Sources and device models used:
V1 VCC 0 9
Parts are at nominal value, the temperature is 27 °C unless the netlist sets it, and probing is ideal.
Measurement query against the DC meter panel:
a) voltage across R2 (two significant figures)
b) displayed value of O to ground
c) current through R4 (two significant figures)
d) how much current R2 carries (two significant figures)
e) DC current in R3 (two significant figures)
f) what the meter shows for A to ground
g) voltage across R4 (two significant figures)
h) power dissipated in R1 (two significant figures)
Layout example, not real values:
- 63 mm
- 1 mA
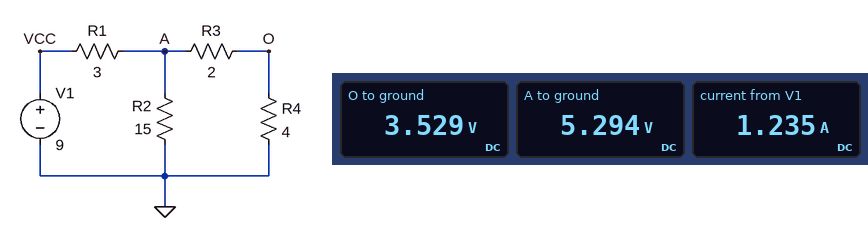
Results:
- 5.3 V
- 3.529 V
- 880 mA
- 350 mA
- 880 mA
- 5.294 V
- 3.5 V
- 4.6 W
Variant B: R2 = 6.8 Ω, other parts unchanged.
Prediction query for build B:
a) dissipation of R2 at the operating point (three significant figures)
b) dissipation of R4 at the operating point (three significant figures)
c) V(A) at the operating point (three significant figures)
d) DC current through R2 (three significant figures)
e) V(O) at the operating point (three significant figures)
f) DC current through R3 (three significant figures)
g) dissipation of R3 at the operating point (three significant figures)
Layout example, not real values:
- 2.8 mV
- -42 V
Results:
- 3.16 W
- 2.39 W
- 4.64 V
- 682 mA
- 3.09 V
- 773 mA
- 1.19 W
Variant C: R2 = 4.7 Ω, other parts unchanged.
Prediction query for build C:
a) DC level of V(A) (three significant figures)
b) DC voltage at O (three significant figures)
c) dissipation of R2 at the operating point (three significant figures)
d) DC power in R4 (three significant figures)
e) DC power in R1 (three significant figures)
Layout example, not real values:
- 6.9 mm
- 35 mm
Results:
- 4.21 V
- 2.81 V
- 3.77 W
- 1.97 W
- 7.65 W
